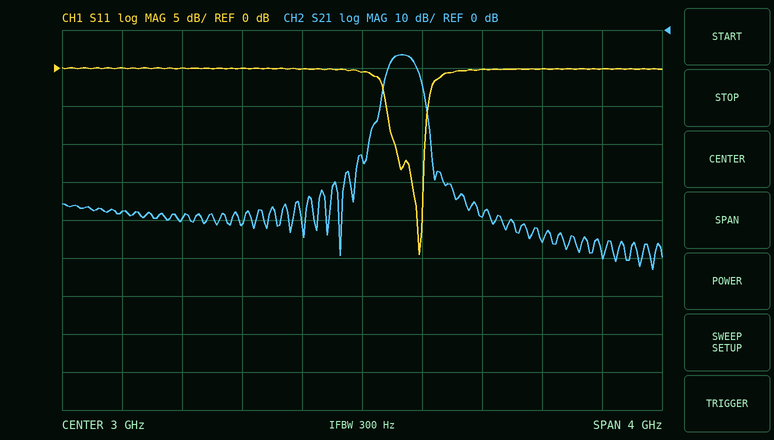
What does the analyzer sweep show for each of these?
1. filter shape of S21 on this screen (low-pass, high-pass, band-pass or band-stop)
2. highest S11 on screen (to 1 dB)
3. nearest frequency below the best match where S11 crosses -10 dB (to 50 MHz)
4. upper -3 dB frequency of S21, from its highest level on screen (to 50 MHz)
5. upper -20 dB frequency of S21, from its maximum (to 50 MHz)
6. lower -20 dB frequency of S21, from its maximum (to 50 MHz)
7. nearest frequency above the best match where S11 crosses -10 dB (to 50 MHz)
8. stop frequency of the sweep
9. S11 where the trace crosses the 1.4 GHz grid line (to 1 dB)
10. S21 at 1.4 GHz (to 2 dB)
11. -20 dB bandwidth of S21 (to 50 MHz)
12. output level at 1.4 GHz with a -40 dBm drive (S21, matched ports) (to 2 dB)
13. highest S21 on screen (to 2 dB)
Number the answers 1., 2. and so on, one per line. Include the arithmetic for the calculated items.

1. band-pass
2. 0 dB
3. 3.20 GHz
4. 3.35 GHz
5. 3.45 GHz
6. 3.05 GHz
7. 3.40 GHz
8. 5 GHz
9. 0 dB
10. -48 dB
11. 3.45 GHz − 3.05 GHz = 400 MHz
12. -40 dBm + (-48 dB) = -88 dBm
13. -6 dB
